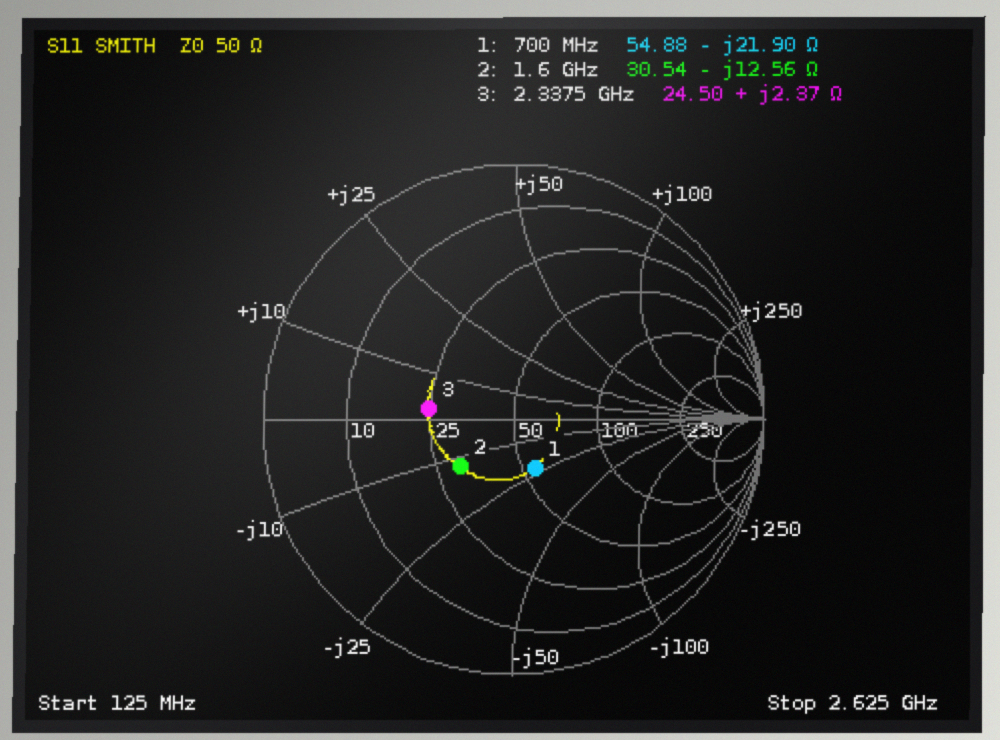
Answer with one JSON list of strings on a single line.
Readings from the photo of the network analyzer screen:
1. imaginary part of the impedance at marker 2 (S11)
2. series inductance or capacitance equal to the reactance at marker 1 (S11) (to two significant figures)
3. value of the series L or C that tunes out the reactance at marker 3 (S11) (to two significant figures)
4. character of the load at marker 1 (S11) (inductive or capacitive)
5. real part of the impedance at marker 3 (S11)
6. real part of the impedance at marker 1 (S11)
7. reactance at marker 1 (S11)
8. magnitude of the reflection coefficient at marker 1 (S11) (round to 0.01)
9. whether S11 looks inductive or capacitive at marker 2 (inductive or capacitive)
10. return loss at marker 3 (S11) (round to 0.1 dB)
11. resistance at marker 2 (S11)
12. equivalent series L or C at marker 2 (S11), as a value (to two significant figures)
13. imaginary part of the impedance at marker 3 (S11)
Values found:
["-12.56 Ω", "10 pF", "29 pF", "capacitive", "24.50 Ω", "54.88 Ω", "-21.90 Ω", "0.21", "capacitive", "9.3 dB", "30.54 Ω", "7.9 pF", "+2.37 Ω"]
